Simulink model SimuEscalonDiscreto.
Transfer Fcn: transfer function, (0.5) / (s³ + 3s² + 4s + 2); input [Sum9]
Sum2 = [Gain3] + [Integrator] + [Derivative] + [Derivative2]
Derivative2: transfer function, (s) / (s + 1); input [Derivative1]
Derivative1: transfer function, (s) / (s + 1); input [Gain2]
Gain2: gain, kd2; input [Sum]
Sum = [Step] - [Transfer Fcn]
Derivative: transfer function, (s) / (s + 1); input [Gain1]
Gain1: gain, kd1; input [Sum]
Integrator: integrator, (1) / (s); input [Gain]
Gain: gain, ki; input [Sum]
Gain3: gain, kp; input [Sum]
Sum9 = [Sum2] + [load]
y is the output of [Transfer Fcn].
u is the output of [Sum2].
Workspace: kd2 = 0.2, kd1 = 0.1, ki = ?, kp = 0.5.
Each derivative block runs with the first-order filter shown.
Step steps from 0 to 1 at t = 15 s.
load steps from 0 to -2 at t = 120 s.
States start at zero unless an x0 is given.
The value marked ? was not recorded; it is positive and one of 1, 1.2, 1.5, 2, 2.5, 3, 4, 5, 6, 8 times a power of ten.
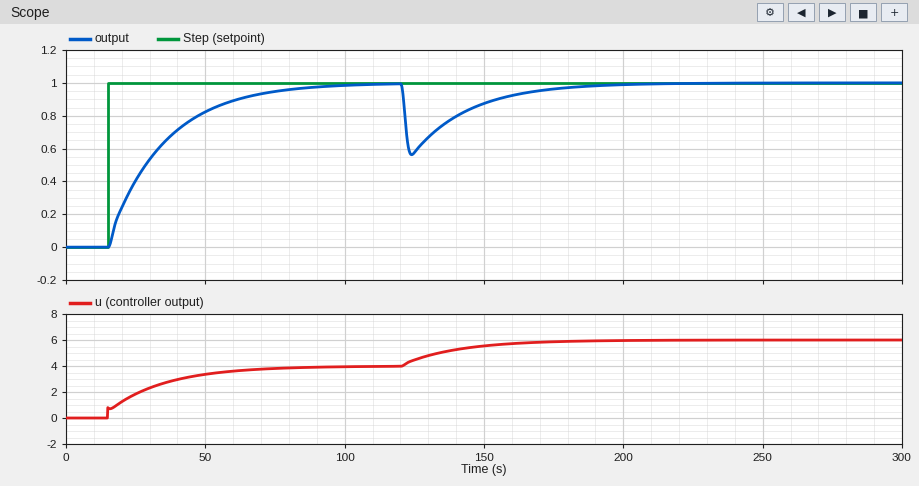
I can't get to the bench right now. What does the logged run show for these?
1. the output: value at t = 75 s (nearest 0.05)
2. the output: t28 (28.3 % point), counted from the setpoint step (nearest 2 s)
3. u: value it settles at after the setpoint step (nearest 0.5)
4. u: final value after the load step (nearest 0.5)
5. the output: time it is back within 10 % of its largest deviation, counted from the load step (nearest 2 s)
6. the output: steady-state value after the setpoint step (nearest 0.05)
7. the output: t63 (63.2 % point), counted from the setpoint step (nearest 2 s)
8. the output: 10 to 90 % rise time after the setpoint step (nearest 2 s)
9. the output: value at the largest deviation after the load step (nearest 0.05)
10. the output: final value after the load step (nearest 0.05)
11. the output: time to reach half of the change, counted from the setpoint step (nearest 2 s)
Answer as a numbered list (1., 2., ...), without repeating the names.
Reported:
1. 0.95
2. 6 s
3. 4.0
4. 6.0
5. 52 s
6. 1.00
7. 20 s
8. 44 s
9. 0.55
10. 1.00
11. 14 s
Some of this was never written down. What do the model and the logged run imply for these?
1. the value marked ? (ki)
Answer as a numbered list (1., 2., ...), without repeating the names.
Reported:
1. 0.2
